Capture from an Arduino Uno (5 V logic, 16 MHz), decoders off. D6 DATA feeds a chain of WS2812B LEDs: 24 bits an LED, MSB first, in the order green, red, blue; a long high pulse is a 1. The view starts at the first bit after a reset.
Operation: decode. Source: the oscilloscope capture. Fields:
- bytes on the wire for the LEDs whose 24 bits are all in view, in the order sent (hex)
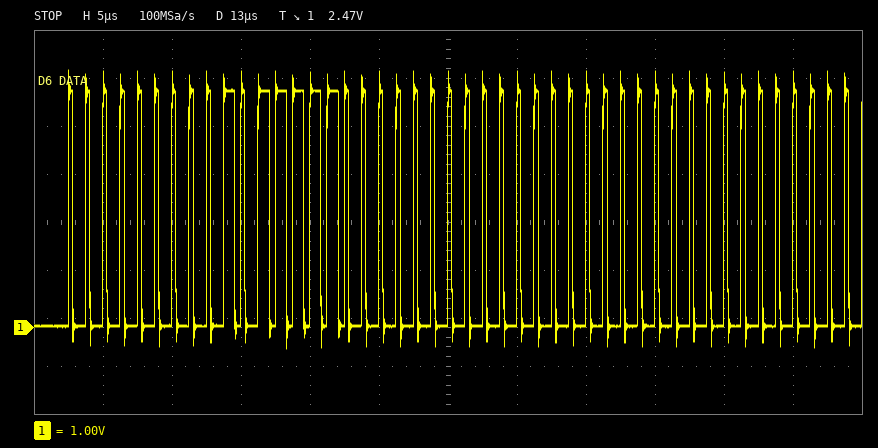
00 5F 00
